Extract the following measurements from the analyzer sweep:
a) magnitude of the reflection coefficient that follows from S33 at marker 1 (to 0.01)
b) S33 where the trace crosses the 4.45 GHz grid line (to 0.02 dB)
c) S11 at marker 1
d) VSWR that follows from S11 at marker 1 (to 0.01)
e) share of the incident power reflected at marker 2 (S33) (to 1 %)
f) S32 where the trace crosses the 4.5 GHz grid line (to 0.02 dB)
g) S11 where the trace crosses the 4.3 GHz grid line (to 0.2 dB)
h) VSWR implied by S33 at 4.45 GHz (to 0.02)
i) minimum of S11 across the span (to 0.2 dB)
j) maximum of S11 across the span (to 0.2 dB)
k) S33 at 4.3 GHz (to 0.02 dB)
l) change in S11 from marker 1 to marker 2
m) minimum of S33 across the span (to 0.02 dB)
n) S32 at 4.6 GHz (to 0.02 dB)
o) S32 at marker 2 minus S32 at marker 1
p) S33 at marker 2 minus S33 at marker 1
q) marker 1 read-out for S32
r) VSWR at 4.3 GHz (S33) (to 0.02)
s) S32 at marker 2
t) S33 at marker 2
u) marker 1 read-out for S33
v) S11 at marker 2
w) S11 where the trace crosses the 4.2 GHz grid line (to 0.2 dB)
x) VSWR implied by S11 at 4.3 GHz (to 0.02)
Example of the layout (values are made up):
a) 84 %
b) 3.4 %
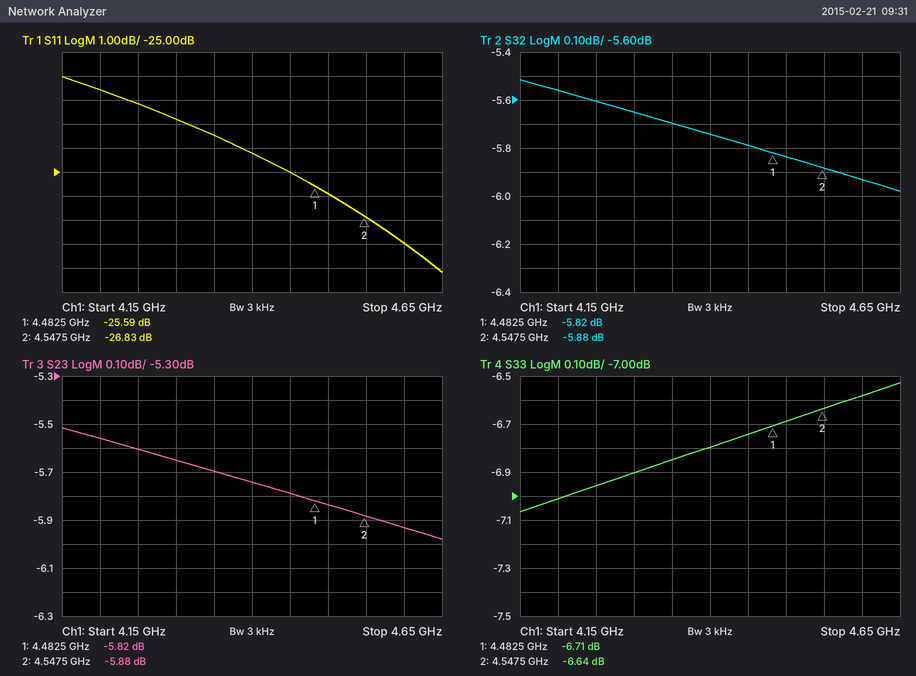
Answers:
a) 0.46
b) -6.74 dB
c) -25.59 dB
d) 1.11
e) 22 %
f) -5.84 dB
g) -22.8 dB
h) 2.70
i) -29.2 dB
j) -21.0 dB
k) -6.90 dB
l) -1.24 dB
m) -7.06 dB
n) -5.94 dB
o) -0.06 dB
p) 0.07 dB
q) -5.82 dB
r) 2.64
s) -5.88 dB
t) -6.64 dB
u) -6.71 dB
v) -26.83 dB
w) -21.6 dB
x) 1.16
